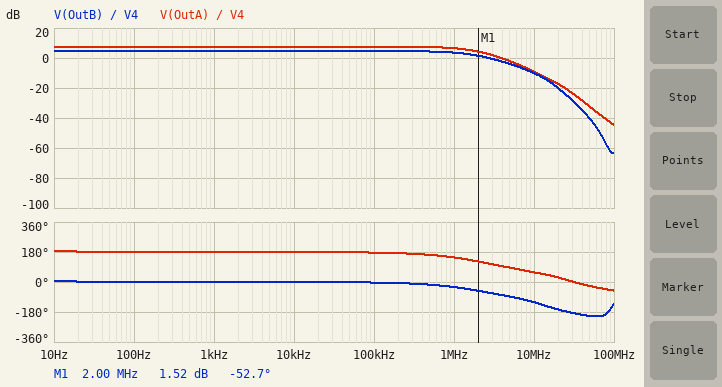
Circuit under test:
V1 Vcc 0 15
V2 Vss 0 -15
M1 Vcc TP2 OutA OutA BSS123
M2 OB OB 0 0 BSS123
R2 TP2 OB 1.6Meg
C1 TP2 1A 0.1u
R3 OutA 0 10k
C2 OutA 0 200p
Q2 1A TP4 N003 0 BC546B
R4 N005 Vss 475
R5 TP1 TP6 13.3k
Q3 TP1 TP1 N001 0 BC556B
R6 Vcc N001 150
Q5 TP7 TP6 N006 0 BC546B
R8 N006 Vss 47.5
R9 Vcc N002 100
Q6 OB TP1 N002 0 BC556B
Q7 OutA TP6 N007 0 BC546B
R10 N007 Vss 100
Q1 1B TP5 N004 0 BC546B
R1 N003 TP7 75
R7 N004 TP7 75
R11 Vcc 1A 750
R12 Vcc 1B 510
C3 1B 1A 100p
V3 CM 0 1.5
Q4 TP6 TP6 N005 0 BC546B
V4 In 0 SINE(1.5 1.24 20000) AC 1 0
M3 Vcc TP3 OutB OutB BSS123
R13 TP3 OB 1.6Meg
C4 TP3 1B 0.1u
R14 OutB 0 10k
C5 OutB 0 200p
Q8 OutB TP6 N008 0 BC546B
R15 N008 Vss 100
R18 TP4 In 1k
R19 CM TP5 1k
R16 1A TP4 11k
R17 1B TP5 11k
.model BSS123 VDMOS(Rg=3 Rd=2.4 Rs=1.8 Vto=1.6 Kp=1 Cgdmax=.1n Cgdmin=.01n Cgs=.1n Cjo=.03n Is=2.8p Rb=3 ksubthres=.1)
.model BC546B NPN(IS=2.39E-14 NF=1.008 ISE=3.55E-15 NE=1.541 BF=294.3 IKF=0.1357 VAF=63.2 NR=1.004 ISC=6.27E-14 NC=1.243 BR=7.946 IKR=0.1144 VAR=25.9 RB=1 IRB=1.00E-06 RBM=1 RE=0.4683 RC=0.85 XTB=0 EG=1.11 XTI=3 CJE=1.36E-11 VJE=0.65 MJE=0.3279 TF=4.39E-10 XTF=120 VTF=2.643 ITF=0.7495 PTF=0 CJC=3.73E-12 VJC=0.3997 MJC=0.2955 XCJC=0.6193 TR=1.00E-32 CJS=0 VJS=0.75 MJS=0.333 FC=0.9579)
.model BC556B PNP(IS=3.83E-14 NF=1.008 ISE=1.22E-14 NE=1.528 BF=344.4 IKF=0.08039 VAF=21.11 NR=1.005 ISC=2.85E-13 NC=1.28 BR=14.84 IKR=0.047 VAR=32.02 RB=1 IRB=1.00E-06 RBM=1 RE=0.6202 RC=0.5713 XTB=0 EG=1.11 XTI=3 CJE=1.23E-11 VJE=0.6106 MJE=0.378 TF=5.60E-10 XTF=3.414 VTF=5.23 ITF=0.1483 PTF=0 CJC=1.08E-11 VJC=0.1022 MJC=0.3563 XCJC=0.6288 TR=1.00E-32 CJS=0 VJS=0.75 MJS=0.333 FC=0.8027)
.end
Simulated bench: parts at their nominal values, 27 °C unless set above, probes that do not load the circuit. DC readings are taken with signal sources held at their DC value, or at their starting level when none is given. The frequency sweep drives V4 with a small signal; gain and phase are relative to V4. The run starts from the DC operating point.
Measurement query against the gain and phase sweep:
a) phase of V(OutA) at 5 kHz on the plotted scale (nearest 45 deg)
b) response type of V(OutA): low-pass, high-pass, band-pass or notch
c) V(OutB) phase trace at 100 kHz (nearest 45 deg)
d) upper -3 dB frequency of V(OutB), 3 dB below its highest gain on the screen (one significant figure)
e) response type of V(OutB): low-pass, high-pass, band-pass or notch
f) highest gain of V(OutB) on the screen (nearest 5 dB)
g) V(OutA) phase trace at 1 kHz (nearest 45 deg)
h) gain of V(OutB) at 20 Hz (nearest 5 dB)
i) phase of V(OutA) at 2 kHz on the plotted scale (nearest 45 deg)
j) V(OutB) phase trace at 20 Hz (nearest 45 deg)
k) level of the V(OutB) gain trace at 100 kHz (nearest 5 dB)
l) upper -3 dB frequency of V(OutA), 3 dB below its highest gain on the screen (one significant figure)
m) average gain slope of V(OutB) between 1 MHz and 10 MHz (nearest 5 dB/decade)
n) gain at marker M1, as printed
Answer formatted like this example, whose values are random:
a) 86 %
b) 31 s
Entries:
a) 180 deg
b) low-pass
c) 0 deg
d) 2 MHz
e) low-pass
f) 5 dB
g) 180 deg
h) 5 dB
i) 180 deg
j) 0 deg
k) 5 dB
l) 2 MHz
m) -15 dB/decade
n) 1.52 dB
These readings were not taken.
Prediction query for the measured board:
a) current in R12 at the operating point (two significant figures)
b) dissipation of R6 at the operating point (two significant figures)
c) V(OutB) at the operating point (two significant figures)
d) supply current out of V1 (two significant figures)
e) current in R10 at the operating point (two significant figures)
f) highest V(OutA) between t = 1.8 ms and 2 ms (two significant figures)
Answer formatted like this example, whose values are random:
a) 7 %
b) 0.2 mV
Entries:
a) 10 mA
b) 640 µW
c) -95 mV
d) 42 mA
e) 8.9 mA
f) 2.9 V
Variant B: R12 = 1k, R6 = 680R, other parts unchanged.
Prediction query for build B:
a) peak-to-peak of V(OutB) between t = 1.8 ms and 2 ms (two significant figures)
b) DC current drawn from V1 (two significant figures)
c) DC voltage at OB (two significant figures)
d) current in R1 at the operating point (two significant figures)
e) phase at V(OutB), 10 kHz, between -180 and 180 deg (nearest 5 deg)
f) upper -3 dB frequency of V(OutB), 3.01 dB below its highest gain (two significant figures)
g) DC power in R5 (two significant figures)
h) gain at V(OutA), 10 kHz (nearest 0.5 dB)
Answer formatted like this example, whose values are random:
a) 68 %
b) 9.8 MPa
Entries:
a) 7.0 V
b) 50 mA
c) 1.8 V
d) 9.3 mA
e) 0 deg
f) 1.6 MHz
g) 53 mW
h) 6.5 dB
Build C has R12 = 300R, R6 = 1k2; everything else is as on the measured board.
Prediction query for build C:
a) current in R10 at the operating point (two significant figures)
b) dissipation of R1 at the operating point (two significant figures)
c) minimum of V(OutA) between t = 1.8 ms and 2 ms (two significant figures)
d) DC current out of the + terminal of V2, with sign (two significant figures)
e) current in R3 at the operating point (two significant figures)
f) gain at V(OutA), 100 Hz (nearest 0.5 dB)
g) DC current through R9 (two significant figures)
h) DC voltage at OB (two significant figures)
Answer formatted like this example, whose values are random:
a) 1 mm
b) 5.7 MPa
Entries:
a) 8.3 mA
b) 3.8 mW
c) -3.0 V
d) -35 mA
e) 12 µA
f) 8.0 dB
g) 22 mA
h) 1.8 V
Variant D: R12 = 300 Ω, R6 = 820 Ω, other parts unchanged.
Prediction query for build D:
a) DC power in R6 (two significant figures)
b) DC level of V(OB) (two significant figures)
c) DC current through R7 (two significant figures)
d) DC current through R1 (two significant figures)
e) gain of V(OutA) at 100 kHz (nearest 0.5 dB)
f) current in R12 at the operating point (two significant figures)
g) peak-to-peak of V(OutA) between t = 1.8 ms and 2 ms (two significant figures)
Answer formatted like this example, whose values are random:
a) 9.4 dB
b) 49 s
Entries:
a) 3.1 mW
b) 1.8 V
c) 10 mA
d) 7.3 mA
e) 8.0 dB
f) 11 mA
g) 6.3 V
